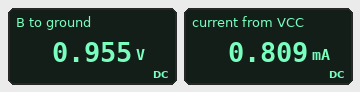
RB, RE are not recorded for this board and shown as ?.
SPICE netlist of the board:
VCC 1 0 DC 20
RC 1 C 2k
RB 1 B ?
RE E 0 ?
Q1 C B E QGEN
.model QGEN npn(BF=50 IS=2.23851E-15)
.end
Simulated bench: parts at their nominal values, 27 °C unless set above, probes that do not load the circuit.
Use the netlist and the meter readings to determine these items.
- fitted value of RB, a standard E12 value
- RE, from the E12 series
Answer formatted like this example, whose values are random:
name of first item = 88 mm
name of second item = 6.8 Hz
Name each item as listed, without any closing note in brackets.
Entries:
fitted value of RB, a standard E12 value = 1.2 MΩ
RE, from the E12 series = 330 Ω
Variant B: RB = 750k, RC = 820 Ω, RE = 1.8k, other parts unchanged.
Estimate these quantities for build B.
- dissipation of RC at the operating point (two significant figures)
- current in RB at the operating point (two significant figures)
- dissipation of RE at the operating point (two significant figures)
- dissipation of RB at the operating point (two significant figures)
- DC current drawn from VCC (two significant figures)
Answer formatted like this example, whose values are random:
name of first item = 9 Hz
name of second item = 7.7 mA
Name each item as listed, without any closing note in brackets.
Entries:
dissipation of RC at the operating point = 1.1 mW
current in RB at the operating point = 23 µA
dissipation of RE at the operating point = 2.5 mW
dissipation of RB at the operating point = 390 µW
DC current drawn from VCC = 1.2 mA
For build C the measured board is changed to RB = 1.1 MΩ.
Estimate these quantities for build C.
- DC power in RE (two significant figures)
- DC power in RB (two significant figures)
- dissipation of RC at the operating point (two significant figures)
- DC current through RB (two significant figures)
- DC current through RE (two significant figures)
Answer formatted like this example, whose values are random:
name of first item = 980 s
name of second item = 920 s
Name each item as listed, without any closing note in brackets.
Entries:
DC power in RE = 260 µW
DC power in RB = 330 µW
dissipation of RC at the operating point = 1.5 mW
DC current through RB = 17 µA
DC current through RE = 880 µA
